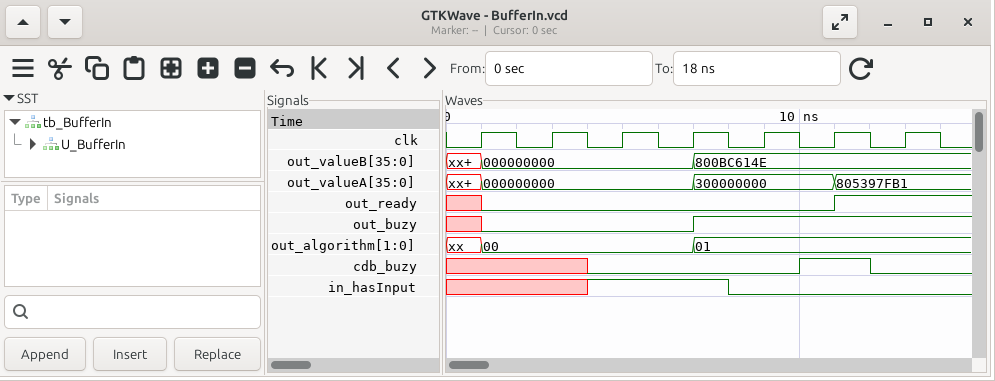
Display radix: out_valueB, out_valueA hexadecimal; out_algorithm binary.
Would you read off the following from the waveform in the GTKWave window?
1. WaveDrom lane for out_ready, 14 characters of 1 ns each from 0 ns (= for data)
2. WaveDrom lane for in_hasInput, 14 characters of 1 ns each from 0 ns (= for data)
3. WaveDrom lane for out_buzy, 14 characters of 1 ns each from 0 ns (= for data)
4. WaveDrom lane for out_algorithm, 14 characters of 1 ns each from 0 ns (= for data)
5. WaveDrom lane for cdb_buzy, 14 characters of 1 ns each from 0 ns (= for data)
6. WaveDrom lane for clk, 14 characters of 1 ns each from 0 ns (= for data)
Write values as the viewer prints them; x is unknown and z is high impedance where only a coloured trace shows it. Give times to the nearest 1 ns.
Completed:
{name: 'out_ready', wave: 'x0.........1..'}
{name: 'in_hasInput', wave: 'x...1...0.....'}
{name: 'out_buzy', wave: 'x0.....1......'}
{name: 'out_algorithm', wave: 'x=.....=......', data: '00 01'}
{name: 'cdb_buzy', wave: 'x...0.....1.0.'}
{name: 'clk', wave: '01010101010101'}
